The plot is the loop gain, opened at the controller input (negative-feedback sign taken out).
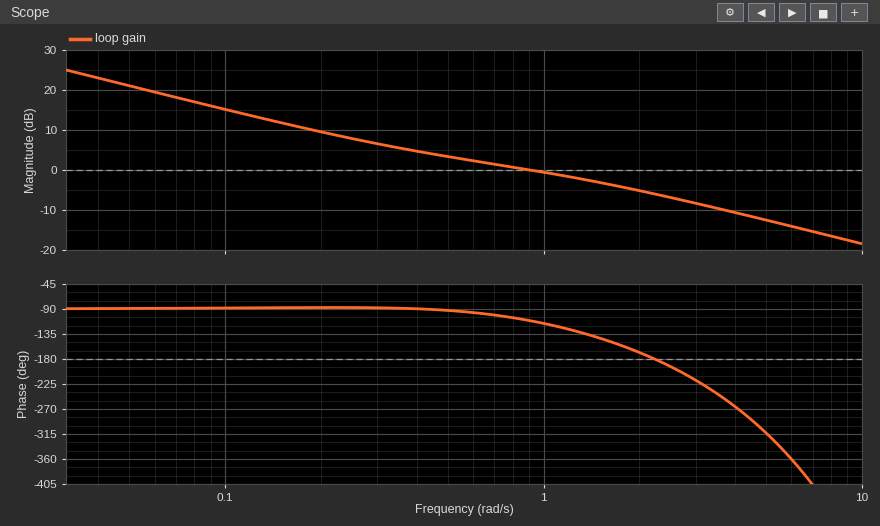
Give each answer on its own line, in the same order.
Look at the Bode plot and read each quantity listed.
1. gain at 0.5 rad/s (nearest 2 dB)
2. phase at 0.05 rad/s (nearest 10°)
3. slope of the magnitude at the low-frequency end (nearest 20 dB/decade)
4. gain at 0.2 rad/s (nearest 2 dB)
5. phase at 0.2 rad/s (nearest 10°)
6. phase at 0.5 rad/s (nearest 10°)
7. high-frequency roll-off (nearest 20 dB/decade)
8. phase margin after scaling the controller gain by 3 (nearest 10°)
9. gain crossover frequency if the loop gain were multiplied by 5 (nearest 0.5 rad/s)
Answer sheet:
4 dB
-90°
-20 dB/decade
10 dB
-90°
-90°
-20 dB/decade
-60°
6.0 rad/s
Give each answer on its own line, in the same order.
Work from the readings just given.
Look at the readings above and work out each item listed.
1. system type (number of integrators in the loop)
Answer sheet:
1
